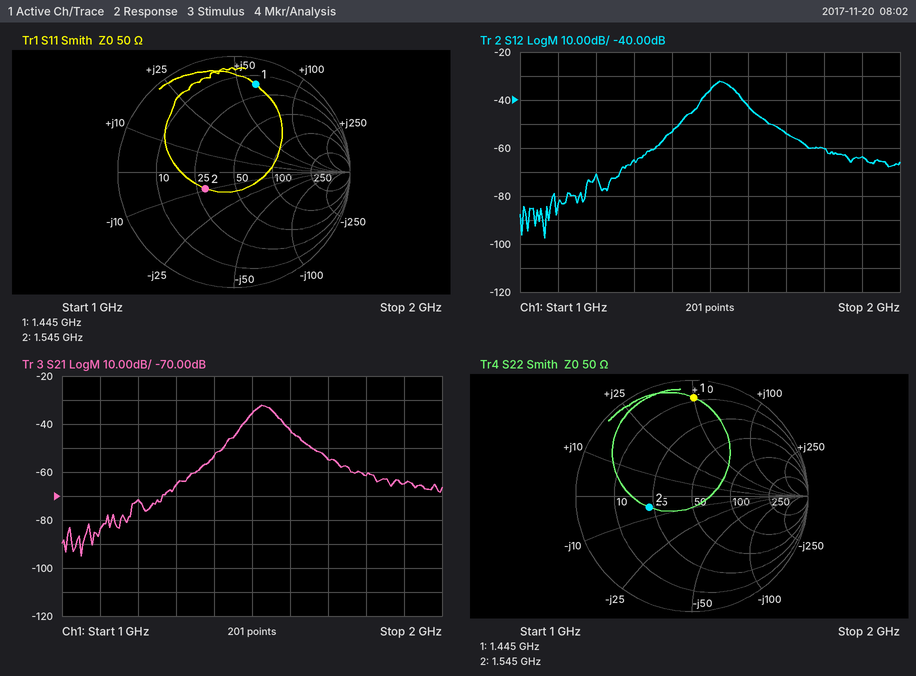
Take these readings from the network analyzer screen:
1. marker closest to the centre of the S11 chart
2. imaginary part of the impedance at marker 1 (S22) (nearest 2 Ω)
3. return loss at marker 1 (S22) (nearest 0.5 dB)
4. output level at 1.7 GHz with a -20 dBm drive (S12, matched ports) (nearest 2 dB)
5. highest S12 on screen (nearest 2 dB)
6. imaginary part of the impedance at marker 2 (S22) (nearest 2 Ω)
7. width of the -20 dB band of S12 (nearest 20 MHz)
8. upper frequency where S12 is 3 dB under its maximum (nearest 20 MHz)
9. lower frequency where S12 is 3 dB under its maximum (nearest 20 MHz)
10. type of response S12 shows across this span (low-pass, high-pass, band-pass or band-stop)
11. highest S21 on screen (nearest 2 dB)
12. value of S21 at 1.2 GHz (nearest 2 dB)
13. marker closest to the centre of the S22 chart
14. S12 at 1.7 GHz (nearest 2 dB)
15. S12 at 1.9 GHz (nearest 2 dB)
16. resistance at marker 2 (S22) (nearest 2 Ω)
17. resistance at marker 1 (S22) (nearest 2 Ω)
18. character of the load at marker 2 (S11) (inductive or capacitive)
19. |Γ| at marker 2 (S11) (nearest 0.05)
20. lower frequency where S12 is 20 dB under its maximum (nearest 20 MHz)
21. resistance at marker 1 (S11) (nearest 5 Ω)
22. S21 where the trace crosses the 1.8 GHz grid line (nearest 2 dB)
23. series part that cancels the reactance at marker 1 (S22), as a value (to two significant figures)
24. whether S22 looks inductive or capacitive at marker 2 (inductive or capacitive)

marker 2
+50 Ω
1.5 dB
-74 dBm
-32 dB
-6 Ω
280 MHz
1.56 GHz
1.50 GHz
band-pass
-32 dB
-72 dB
marker 2
-54 dB
-64 dB
22 Ω
8 Ω
capacitive
0.30
1.40 GHz
15 Ω
-62 dB
2.2 pF
capacitive
